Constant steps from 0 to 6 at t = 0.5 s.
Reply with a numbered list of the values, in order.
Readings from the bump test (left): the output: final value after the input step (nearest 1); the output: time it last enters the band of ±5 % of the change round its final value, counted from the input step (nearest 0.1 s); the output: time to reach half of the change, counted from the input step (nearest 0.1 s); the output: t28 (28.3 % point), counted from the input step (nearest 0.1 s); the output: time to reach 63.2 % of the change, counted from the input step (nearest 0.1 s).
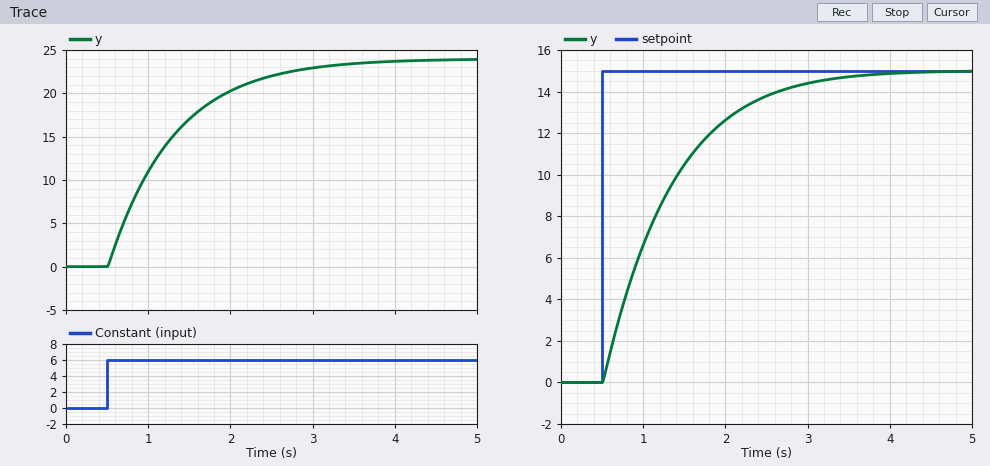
1. 24
2. 2.4 s
3. 0.6 s
4. 0.3 s
5. 0.8 s
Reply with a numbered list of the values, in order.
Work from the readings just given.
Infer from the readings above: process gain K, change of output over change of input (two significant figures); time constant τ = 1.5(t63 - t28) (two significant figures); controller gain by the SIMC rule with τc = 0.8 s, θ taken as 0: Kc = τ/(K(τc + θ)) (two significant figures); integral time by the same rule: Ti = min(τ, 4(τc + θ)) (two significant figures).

1. 4.0
2. 0.75 s
3. 0.23
4. 0.75 s
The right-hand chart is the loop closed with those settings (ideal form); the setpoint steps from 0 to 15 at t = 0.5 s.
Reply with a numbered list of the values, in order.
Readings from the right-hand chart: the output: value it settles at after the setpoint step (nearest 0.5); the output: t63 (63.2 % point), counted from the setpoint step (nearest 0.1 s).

1. 15.0
2. 0.8 s
